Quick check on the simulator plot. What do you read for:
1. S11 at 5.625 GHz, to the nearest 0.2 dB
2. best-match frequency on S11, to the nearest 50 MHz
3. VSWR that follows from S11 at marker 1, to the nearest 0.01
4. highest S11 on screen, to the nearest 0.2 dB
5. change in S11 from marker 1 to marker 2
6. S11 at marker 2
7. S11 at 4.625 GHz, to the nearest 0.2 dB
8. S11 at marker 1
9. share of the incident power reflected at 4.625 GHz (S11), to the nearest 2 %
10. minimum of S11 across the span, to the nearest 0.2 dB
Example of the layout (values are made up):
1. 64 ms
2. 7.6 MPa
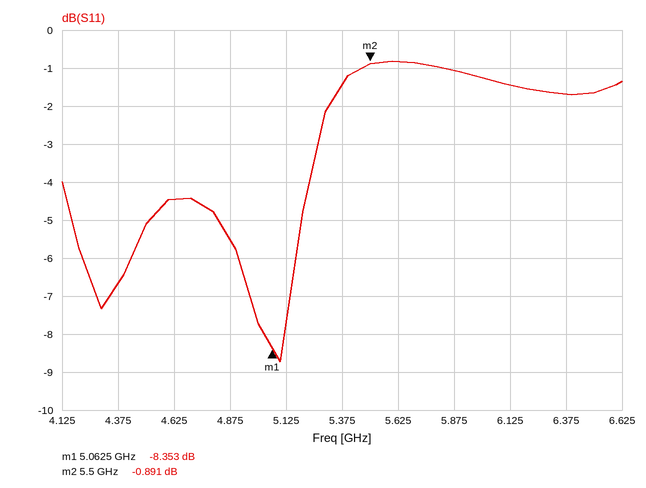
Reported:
1. -0.8 dB
2. 5.10 GHz
3. 2.24
4. -0.8 dB
5. 7.462 dB
6. -0.891 dB
7. -4.4 dB
8. -8.353 dB
9. 36 %
10. -8.8 dB
